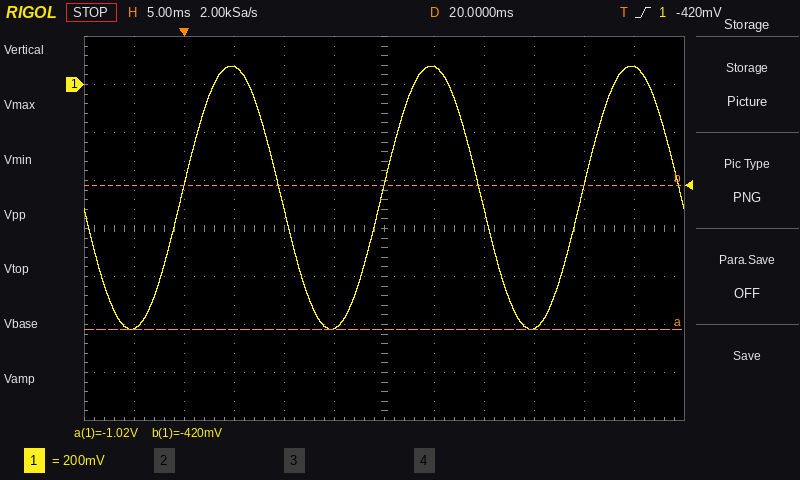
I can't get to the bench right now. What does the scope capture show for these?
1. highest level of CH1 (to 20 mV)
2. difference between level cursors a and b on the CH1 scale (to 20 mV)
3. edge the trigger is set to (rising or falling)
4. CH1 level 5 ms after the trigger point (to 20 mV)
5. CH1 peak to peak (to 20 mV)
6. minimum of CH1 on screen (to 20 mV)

80 mV
600 mV
rising
80 mV
1.10 V
-1.02 V
